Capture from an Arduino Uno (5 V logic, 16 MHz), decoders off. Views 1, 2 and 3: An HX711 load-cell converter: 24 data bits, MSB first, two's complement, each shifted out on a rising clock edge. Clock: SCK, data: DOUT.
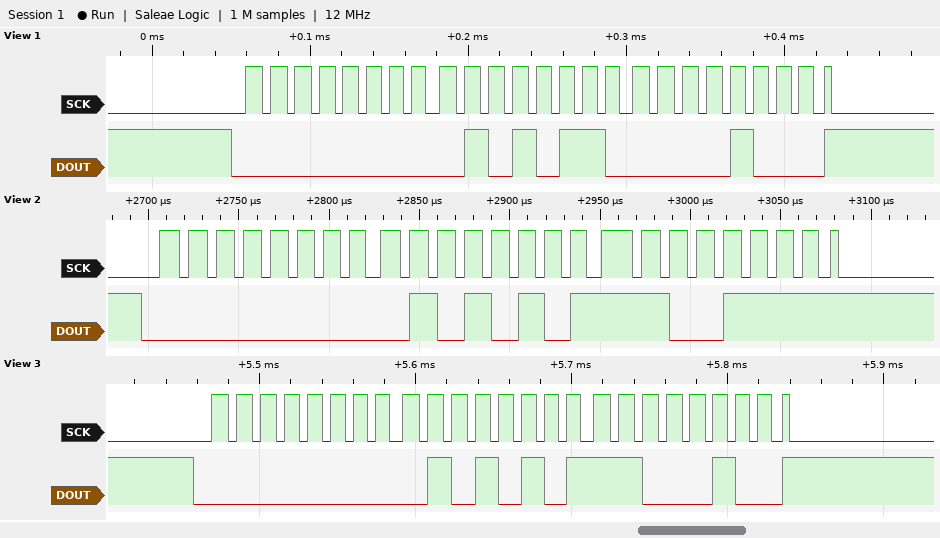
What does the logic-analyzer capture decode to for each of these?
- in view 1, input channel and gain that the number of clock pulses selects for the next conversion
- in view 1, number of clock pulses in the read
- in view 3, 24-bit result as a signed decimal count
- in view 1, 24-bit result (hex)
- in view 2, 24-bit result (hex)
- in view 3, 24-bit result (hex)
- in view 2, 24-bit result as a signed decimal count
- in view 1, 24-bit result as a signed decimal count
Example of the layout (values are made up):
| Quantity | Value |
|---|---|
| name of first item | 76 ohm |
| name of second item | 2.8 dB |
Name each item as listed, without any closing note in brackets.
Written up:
| Quantity | Value |
|---|---|
| in view 1, input channel and gain that the number of clock pulses selects for the next conversion | channel A, gain 128 |
| in view 1, number of clock pulses in the read | 25 |
| in view 3, 24-bit result as a signed decimal count | 21956 |
| in view 1, 24-bit result | 0x005608 |
| in view 2, 24-bit result | 0x0055CF |
| in view 3, 24-bit result | 0x0055C4 |
| in view 2, 24-bit result as a signed decimal count | 21967 |
| in view 1, 24-bit result as a signed decimal count | 22024 |
